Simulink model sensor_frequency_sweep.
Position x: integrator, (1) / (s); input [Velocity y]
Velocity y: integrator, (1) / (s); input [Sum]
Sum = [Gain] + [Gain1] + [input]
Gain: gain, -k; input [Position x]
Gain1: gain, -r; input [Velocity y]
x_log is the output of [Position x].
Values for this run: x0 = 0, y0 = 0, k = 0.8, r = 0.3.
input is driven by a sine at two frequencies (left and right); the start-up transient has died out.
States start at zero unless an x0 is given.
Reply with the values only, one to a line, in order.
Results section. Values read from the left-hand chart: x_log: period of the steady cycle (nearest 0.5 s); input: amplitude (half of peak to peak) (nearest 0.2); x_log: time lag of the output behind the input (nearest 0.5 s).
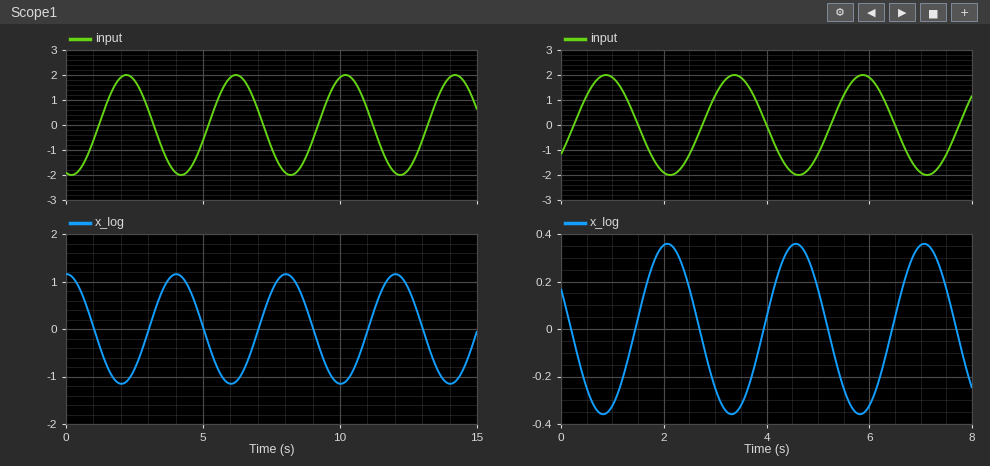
4.0 s
2.0
2.0 s
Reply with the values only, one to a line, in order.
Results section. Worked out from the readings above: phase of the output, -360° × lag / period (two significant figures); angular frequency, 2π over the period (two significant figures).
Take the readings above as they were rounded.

-180°
1.6 rad/s
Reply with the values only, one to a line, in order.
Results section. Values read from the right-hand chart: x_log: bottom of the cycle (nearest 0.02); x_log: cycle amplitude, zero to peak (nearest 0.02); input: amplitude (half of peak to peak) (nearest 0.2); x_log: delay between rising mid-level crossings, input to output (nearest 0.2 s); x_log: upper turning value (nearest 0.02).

-0.36
0.36
2.0
1.2 s
0.36
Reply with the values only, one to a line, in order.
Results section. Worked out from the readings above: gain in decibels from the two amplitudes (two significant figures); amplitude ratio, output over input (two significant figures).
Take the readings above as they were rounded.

-15 dB
0.18
